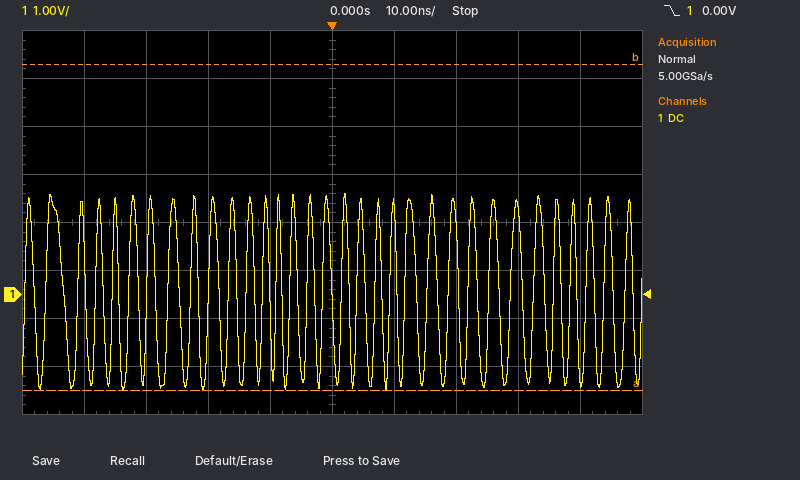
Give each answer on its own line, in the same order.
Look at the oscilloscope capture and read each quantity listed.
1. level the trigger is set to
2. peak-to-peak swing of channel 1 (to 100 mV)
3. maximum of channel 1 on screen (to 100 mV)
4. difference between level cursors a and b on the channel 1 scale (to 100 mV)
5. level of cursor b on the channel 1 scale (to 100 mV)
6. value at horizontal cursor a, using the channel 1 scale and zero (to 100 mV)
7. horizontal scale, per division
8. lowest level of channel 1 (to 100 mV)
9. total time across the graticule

0.00 V
4.1 V
2.1 V
6.8 V
4.8 V
-2.0 V
10 ns
-2.0 V
100 ns
